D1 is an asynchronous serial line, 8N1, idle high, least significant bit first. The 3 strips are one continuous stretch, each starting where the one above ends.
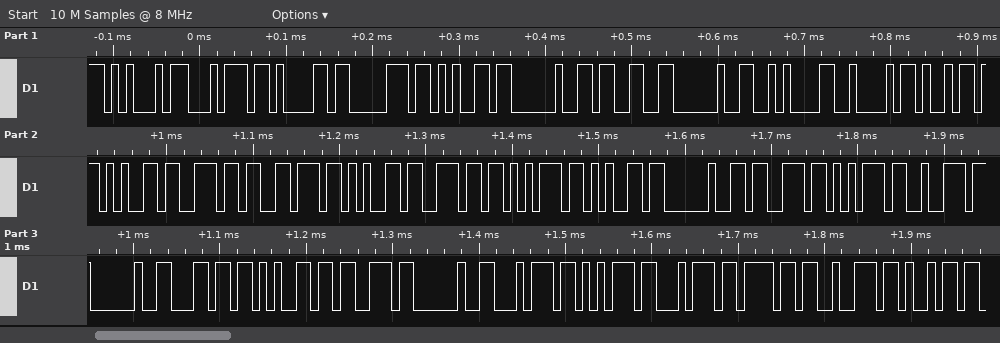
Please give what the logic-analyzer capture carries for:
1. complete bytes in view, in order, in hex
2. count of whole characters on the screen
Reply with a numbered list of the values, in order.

1. 45 74 61 70 65 20 33 20 0A 42 69 65 6E 76 65 6E 75 65 20 73 75 72 20 6C 65 73 20 74 75 74 6F 72 69
2. 33
